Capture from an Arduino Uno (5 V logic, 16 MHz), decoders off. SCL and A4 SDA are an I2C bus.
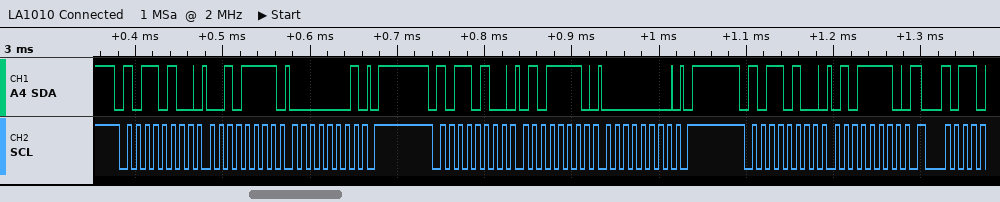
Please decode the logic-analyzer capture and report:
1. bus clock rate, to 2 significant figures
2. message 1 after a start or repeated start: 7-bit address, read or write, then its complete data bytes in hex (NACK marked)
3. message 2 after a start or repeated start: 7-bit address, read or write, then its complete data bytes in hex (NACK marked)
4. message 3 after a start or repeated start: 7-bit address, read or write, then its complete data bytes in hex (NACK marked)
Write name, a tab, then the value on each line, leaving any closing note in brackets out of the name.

bus clock rate, to 2 significant figures	100 kHz
message 1 after a start or repeated start: 7-bit address, read or write, then its complete data bytes in hex	0x5A write: 2F 01
message 2 after a start or repeated start: 7-bit address, read or write, then its complete data bytes in hex	0x5A write: 5E 00
message 3 after a start or repeated start: 7-bit address, read or write, then its complete data bytes in hex	0x5A write: 5E
